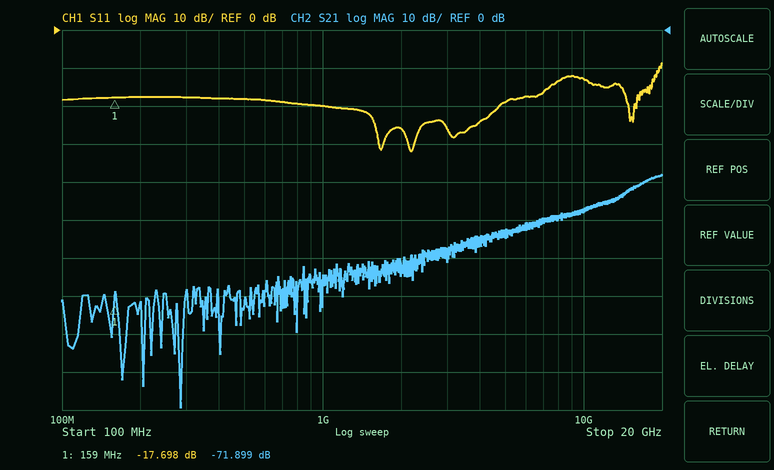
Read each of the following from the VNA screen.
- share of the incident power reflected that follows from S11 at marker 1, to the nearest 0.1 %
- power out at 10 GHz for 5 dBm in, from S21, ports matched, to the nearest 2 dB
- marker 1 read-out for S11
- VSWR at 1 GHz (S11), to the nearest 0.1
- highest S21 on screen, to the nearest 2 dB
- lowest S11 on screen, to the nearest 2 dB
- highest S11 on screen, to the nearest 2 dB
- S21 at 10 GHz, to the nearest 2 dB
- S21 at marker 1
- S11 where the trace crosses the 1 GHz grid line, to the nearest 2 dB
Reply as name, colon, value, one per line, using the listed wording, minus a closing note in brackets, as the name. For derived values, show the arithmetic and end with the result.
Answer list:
share of the incident power reflected that follows from S11 at marker 1, to the nearest 0.1 %: 10^(-17.698/10) ≈ 1.7 %
power out at 10 GHz for 5 dBm in, from S21, ports matched, to the nearest 2 dB: 5 dBm + (-48 dB) = -42 dBm
marker 1 read-out for S11: -17.698 dB
VSWR at 1 GHz (S11), to the nearest 0.1: |Γ| = 10^(-20/20) = 0.1000; VSWR = (1 + 0.1000)/(1 − 0.1000) ≈ 1.2
highest S21 on screen, to the nearest 2 dB: -38 dB
lowest S11 on screen, to the nearest 2 dB: -32 dB
highest S11 on screen, to the nearest 2 dB: -8 dB
S21 at 10 GHz, to the nearest 2 dB: -48 dB
S21 at marker 1: -71.899 dB
S11 where the trace crosses the 1 GHz grid line, to the nearest 2 dB: -20 dB
